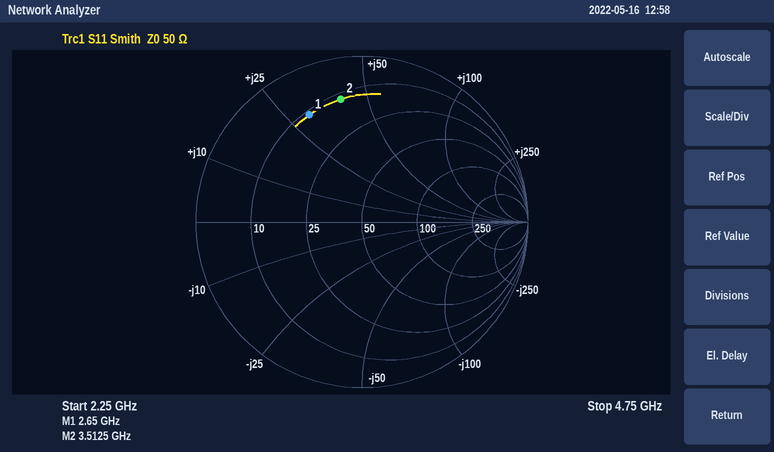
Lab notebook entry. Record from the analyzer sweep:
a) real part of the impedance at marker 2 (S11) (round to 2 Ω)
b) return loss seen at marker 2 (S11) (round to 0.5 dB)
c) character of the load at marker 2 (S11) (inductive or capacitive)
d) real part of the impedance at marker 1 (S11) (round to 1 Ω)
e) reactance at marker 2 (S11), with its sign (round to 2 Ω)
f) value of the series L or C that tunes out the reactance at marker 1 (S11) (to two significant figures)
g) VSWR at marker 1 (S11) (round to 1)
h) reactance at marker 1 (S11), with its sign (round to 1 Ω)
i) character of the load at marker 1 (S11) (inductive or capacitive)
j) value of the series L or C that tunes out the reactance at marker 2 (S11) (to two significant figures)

12 Ω
2.5 dB
inductive
11 Ω
+40 Ω
2.0 pF
6
+30 Ω
inductive
1.1 pF
